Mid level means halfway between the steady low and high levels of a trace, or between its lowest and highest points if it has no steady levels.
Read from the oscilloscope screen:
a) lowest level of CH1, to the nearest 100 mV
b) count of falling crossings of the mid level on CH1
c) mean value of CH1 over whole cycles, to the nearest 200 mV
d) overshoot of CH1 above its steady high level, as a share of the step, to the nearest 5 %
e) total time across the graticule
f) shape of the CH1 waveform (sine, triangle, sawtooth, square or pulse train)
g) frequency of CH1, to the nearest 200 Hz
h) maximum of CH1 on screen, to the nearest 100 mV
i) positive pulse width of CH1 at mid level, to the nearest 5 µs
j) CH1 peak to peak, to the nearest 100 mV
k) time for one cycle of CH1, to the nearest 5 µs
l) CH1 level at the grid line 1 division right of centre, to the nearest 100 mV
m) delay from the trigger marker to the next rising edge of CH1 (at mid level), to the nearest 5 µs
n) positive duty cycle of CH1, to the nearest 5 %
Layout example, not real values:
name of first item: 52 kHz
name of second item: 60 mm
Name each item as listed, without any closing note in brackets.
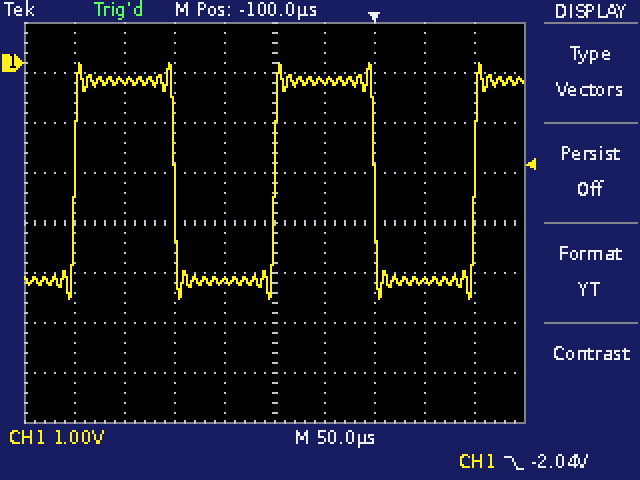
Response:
lowest level of CH1, to the nearest 100 mV: -4.7 V
count of falling crossings of the mid level on CH1: 2
mean value of CH1 over whole cycles, to the nearest 200 mV: -2.4 V
overshoot of CH1 above its steady high level, as a share of the step, to the nearest 5 %: 10 %
total time across the graticule: 500 µs
shape of the CH1 waveform: square
frequency of CH1, to the nearest 200 Hz: 5.0 kHz
maximum of CH1 on screen, to the nearest 100 mV: 0.0 V
positive pulse width of CH1 at mid level, to the nearest 5 µs: 100 µs
CH1 peak to peak, to the nearest 100 mV: 4.7 V
time for one cycle of CH1, to the nearest 5 µs: 200 µs
CH1 level at the grid line 1 division right of centre, to the nearest 100 mV: -400 mV
delay from the trigger marker to the next rising edge of CH1 (at mid level), to the nearest 5 µs: 100 µs
positive duty cycle of CH1, to the nearest 5 %: 50 %
